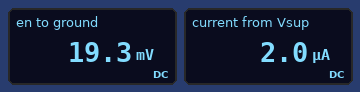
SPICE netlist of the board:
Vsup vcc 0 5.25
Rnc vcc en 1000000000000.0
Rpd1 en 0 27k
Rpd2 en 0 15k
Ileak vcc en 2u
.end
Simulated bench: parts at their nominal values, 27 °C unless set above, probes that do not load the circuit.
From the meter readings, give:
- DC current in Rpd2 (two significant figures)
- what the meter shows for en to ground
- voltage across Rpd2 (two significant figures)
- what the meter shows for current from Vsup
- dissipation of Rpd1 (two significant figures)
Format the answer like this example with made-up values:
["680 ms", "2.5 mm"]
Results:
["1.3 µA", "19.3 mV", "19 mV", "2.0 µA", "14 nW"]
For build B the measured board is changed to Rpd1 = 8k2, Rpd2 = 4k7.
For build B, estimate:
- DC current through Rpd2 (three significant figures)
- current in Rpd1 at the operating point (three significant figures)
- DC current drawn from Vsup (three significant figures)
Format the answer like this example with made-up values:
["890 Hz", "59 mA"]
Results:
["1.27 µA", "729 nA", "2.00 µA"]
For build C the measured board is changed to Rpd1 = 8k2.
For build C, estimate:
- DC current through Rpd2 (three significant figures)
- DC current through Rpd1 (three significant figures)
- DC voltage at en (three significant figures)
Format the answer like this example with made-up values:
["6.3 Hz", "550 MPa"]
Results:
["707 nA", "1.29 µA", "10.6 mV"]
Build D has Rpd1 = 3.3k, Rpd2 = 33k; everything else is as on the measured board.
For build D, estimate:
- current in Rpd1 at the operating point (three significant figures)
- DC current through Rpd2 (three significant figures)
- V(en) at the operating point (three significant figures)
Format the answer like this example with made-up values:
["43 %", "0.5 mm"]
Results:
["1.82 µA", "182 nA", "6.00 mV"]
